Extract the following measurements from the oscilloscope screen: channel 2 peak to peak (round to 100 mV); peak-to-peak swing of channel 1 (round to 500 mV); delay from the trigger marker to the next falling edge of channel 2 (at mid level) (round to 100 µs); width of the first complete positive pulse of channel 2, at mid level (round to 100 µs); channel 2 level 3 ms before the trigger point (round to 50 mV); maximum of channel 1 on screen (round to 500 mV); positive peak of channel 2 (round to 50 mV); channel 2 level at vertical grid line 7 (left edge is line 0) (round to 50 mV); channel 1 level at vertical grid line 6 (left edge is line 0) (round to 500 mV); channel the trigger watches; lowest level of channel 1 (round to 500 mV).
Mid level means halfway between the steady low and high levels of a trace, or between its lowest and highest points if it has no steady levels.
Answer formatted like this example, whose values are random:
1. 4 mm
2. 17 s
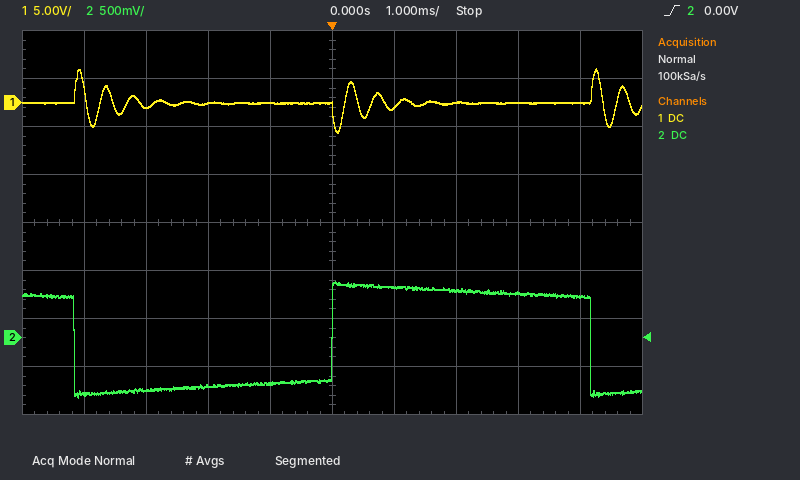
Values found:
1. 1.20 V
2. 6.5 V
3. 4.2 ms
4. 4.2 ms
5. -550 mV
6. 3.5 V
7. 600 mV
8. 500 mV
9. -500 mV
10. channel 2
11. -3.0 V
